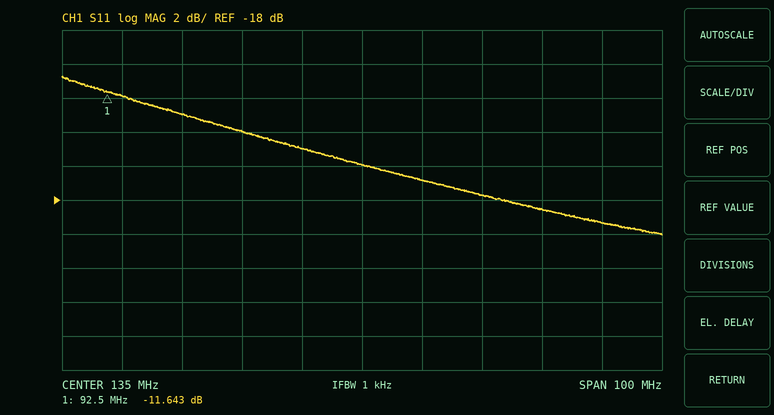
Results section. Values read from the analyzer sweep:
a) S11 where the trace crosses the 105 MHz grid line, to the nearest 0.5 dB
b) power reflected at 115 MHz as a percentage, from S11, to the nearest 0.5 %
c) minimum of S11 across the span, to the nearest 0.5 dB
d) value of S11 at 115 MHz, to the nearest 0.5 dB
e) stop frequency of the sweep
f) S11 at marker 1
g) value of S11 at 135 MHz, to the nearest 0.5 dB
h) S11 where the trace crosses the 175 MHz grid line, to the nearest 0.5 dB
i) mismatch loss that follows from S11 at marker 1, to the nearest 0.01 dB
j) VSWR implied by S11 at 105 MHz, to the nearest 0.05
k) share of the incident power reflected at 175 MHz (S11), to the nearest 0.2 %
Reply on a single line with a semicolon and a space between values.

-13.0 dB; 4.0 %; -20.0 dB; -14.0 dB; 185 MHz; -11.643 dB; -16.0 dB; -19.5 dB; 0.31 dB; 1.60; 1.2 %
